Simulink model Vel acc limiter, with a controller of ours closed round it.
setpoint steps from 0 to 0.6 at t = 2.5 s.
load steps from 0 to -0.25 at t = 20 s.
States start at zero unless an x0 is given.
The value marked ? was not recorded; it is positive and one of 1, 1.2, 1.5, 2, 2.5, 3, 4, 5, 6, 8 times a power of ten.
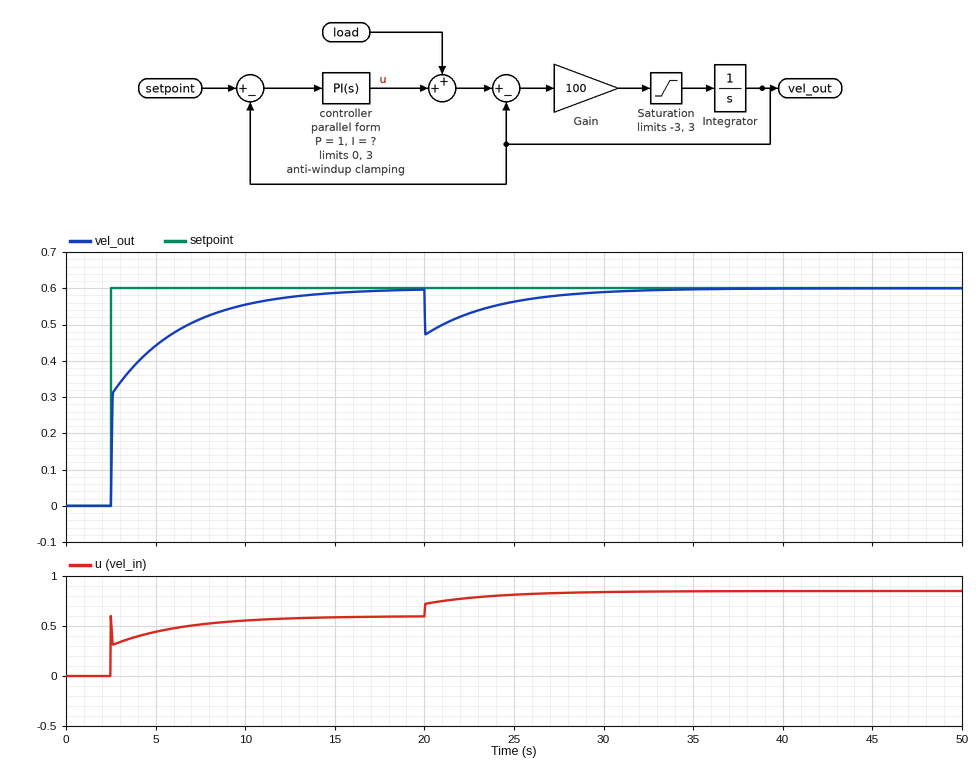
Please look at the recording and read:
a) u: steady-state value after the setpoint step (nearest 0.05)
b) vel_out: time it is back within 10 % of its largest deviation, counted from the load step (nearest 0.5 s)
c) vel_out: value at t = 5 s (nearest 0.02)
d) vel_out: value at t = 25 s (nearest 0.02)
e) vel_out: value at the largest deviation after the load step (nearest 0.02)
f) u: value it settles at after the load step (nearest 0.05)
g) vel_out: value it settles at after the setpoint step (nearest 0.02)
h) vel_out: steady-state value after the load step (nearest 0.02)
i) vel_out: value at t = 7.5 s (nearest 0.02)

0.60
9.5 s
0.44
0.56
0.48
0.85
0.60
0.60
0.52
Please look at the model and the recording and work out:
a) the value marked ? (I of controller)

0.5
